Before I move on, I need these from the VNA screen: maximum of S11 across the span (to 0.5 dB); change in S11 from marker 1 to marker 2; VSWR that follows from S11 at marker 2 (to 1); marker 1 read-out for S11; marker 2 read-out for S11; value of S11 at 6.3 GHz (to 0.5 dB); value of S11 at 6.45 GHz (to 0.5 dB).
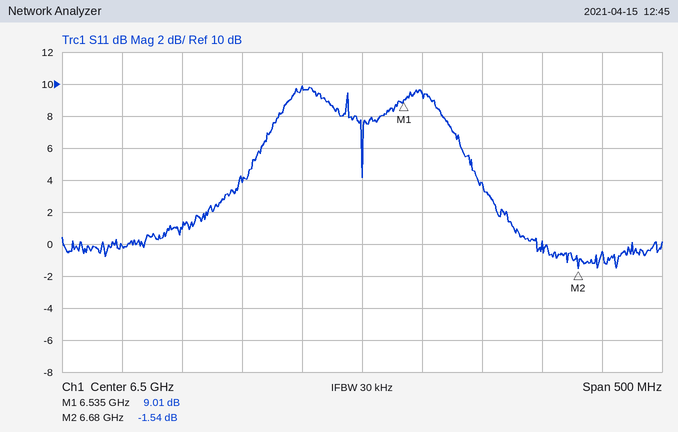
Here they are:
10.0 dB
-10.55 dB
11
9.01 dB
-1.54 dB
0.0 dB
10.0 dB
